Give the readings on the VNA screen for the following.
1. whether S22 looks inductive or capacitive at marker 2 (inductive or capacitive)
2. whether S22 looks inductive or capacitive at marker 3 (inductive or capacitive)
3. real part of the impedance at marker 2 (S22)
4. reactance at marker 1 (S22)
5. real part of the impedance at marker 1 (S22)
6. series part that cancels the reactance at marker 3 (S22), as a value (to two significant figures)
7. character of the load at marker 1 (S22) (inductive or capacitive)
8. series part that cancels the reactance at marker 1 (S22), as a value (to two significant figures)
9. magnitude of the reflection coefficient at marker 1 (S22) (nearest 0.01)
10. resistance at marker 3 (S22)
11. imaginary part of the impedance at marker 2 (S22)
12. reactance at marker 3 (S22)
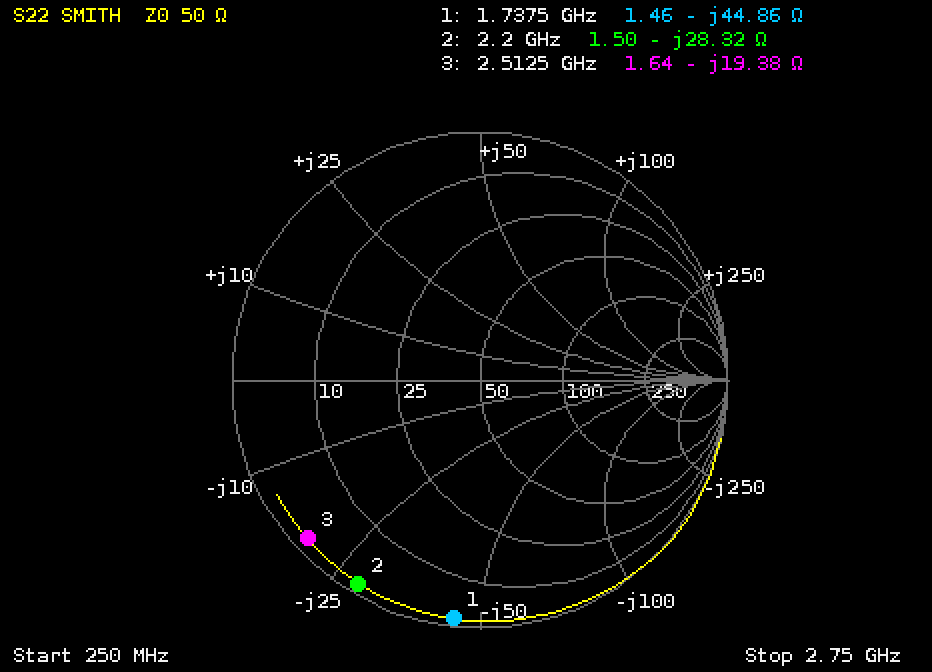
capacitive
capacitive
1.50 Ω
-44.86 Ω
1.46 Ω
1.2 nH
capacitive
4.1 nH
0.97
1.64 Ω
-28.32 Ω
-19.38 Ω
